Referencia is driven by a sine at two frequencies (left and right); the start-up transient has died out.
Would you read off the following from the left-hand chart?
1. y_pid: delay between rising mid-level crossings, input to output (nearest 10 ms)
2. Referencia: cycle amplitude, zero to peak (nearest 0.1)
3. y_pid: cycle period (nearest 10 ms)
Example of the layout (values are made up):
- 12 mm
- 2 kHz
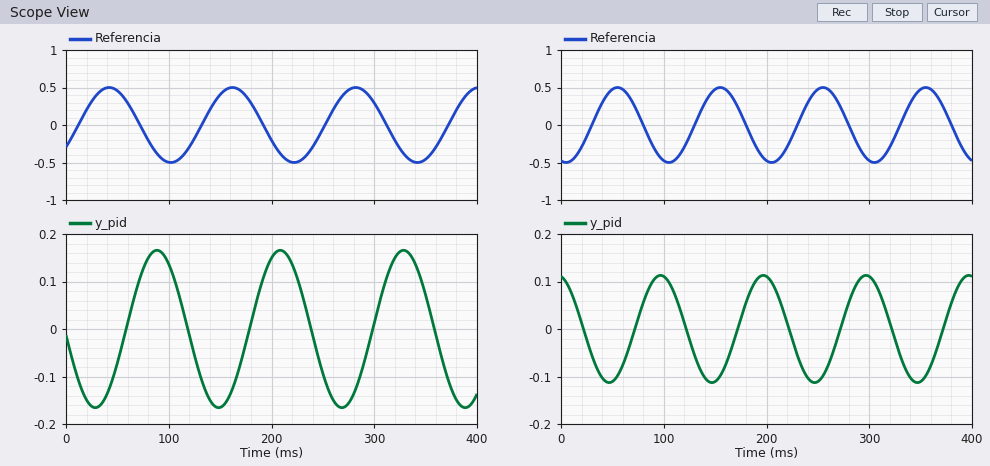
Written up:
- 50 ms
- 0.5
- 120 ms
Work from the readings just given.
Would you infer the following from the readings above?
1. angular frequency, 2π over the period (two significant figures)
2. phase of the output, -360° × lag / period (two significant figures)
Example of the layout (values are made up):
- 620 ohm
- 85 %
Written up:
- 0.052 rad/ms
- -150°
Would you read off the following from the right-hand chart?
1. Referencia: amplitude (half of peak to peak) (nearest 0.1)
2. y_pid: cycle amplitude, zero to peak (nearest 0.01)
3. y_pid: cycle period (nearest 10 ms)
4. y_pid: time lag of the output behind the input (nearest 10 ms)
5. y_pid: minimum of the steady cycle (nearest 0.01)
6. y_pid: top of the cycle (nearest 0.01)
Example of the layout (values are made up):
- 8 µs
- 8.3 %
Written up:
- 0.5
- 0.11
- 100 ms
- 40 ms
- -0.11
- 0.11
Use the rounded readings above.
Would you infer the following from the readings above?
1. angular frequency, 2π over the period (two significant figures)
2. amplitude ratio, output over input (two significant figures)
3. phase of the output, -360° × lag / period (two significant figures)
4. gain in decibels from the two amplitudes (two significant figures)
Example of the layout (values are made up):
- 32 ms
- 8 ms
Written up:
- 0.063 rad/ms
- 0.22
- -140°
- -13 dB
